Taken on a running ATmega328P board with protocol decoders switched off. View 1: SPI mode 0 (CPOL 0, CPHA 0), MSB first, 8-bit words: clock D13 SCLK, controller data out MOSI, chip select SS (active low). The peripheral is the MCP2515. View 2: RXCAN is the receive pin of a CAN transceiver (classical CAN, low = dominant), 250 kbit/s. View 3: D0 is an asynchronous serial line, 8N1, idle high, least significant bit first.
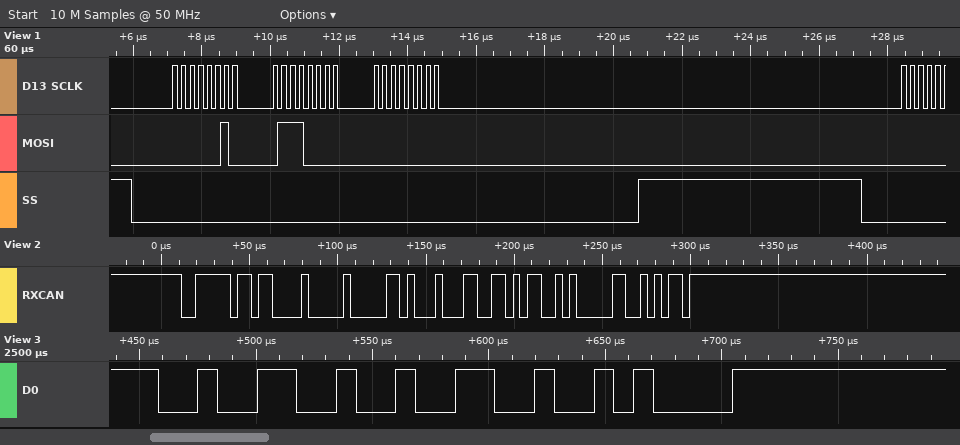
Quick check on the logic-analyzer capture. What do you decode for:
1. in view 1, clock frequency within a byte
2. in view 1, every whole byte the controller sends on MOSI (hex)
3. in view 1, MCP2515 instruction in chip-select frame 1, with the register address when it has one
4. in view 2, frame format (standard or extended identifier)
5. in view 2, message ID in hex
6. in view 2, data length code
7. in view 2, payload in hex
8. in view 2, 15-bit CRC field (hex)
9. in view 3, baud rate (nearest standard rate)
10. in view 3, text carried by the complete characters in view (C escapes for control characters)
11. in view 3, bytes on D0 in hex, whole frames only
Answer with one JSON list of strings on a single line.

["4 MHz", "02 70 00", "WRITE 0x70", "standard", "0x3FB", "4", "00 A2 33 59", "0x2095", "115200 baud", "\"22\\n\"", "0x32 0x32 0x0A"]
